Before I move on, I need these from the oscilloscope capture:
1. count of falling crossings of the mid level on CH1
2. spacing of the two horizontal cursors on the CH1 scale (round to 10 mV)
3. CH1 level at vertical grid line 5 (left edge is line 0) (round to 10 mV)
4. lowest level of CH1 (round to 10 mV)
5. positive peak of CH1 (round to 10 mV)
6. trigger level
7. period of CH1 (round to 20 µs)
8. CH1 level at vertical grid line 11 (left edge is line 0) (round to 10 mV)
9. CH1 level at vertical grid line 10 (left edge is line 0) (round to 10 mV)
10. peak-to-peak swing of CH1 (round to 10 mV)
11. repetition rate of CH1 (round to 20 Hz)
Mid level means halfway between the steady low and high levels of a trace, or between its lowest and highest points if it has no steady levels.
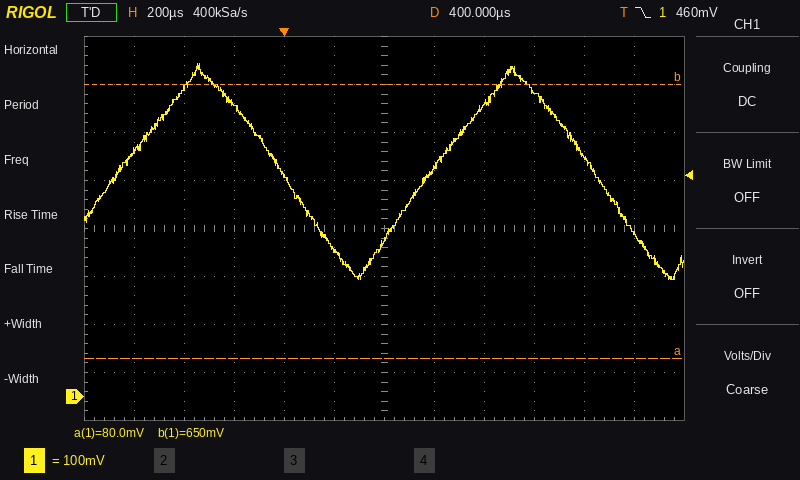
2
570 mV
310 mV
240 mV
690 mV
460 mV
1.26 ms
340 mV
500 mV
450 mV
800 Hz
